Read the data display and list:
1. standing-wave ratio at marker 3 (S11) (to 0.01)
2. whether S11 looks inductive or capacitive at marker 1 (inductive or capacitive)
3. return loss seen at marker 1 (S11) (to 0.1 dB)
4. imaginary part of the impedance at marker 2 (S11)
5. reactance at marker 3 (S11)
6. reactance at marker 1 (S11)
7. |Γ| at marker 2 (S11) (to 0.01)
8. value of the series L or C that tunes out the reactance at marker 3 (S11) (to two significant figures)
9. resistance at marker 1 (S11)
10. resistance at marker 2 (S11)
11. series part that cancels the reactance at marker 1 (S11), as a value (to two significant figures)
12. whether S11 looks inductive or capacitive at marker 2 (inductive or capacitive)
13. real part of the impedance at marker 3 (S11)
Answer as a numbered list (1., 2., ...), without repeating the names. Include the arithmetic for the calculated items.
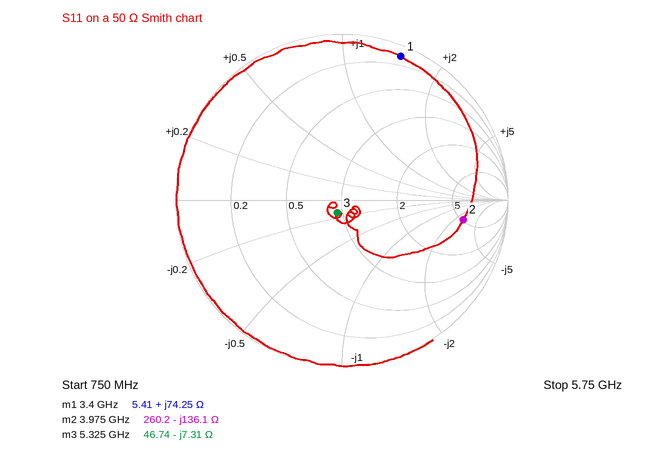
1. 1.18
2. inductive
3. 0.6 dB
4. -136.1 Ω
5. -7.31 Ω
6. +74.25 Ω
7. 0.74
8. L = 7.31 Ω/(2π × 5.325 GHz) ≈ 218 pH, so 220 pH to two significant figures
9. 5.41 Ω
10. 260.2 Ω
11. C = 1/(2π × 3.4 GHz × 74.25 Ω) ≈ 630 fF
12. capacitive
13. 46.74 Ω
